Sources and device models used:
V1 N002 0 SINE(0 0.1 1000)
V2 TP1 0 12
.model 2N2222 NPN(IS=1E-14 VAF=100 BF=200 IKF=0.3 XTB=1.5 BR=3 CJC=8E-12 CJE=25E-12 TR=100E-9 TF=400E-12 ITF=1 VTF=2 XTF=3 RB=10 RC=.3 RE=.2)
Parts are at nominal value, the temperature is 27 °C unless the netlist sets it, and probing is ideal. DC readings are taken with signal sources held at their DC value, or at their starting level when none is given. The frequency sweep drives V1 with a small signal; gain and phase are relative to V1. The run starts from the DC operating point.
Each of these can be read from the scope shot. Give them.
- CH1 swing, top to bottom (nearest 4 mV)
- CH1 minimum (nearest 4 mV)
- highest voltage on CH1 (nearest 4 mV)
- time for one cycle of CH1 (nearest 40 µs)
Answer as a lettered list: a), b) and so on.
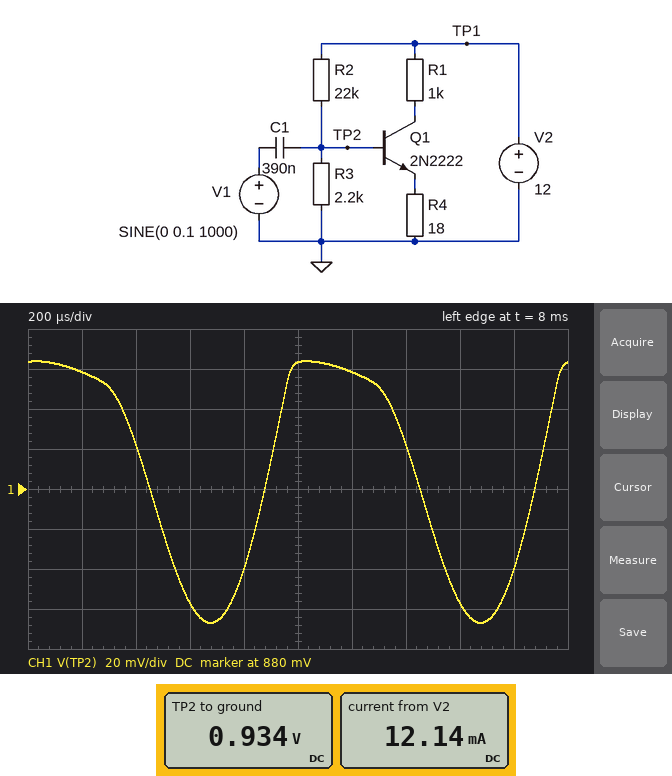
a) 132 mV
b) 812 mV
c) 944 mV
d) 1.00 ms
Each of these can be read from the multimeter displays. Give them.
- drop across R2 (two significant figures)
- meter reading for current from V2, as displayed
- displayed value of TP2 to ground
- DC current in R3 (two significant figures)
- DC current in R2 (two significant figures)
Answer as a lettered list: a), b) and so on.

a) 11 V
b) 12.14 mA
c) 0.934 V
d) 420 µA
e) 500 µA
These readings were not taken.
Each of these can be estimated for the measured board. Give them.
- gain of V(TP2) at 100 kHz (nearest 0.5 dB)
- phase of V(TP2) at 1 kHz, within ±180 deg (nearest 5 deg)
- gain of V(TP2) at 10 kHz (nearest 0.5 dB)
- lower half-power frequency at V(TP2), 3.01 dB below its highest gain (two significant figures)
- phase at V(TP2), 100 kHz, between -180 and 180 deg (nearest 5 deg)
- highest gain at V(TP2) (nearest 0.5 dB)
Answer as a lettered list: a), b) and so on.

a) 0 dB
b) 80 deg
c) -1.5 dB
d) 6.4 kHz
e) 5 deg
f) 0 dB
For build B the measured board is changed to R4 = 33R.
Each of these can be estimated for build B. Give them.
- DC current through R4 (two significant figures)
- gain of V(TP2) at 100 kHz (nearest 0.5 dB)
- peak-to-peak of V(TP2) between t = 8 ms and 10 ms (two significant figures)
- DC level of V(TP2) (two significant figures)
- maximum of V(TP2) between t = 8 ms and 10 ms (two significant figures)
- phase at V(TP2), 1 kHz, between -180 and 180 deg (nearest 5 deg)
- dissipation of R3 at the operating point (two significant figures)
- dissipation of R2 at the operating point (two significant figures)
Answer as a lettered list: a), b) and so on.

a) 8.8 mA
b) 0 dB
c) 190 mV
d) 1.0 V
e) 1.1 V
f) 15 deg
g) 460 µW
h) 5.5 mW
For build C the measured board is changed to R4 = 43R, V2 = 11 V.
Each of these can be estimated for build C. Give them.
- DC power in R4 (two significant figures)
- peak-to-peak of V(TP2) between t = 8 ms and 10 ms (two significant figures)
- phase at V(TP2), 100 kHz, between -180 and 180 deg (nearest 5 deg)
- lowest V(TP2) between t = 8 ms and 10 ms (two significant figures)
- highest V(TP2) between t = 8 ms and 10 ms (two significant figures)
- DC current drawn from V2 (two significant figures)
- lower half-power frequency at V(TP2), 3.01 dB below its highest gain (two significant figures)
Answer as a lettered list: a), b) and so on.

a) 1.4 mW
b) 190 mV
c) 0 deg
d) 850 mV
e) 1.0 V
f) 6.1 mA
g) 250 Hz
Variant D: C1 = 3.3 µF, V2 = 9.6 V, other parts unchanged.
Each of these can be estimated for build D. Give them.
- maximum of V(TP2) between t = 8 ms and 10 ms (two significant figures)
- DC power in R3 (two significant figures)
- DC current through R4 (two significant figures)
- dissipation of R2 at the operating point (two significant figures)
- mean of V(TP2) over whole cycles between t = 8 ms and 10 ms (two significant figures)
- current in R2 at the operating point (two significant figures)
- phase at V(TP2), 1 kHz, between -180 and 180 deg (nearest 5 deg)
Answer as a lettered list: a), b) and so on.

a) 890 mV
b) 300 µW
c) 6.1 mA
d) 3.5 mW
e) 790 mV
f) 400 µA
g) 0 deg
